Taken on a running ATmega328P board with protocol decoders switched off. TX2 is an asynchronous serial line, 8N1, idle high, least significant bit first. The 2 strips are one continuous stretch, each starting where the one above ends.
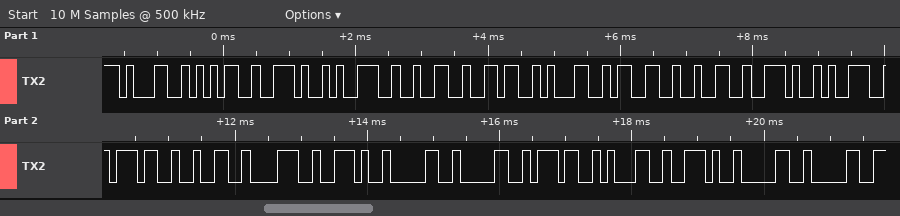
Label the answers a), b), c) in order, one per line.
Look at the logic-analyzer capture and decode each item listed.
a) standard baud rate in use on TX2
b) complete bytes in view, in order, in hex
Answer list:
a) 9600 baud
b) 0x31 0x35 0x2E 0x39 0x32 0x36 0x31 0x33 0x32 0x2E 0x39 0x37 0x32 0x38 0x2E 0x30 0x30 0x37 0x31 0x2E 0x30 0x30
